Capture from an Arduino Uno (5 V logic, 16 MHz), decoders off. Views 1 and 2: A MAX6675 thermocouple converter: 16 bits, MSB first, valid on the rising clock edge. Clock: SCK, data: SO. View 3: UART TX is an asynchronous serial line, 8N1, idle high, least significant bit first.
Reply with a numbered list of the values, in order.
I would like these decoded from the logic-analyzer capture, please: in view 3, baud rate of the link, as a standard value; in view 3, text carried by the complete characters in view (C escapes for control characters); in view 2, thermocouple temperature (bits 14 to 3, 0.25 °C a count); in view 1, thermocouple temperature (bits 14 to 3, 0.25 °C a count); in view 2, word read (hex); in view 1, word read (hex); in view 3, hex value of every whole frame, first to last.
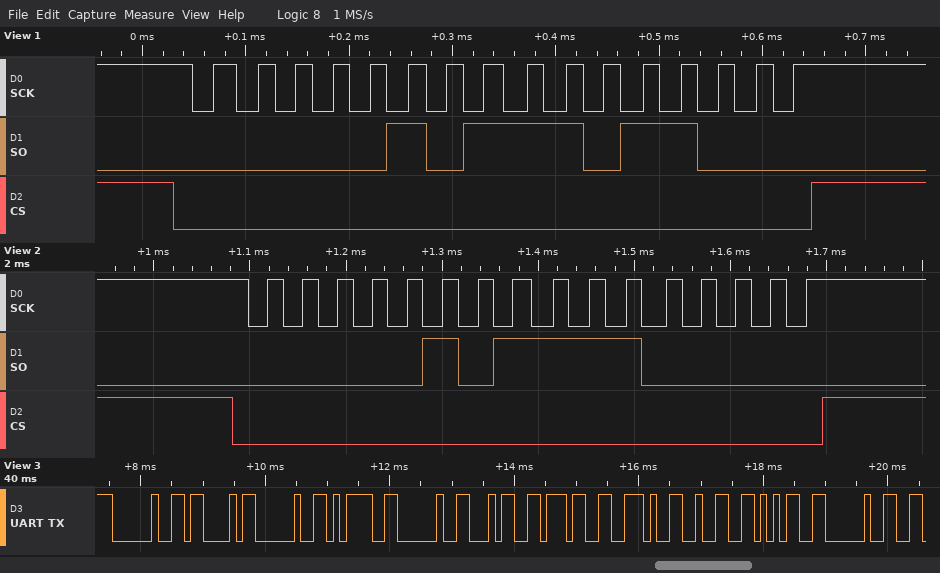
1. 9600 baud
2. " C = 47.25 "
3. 47.00 °C
4. 46.75 °C
5. 0x05E0
6. 0x05D8
7. 20 43 20 3D 20 34 37 2E 32 35 20
